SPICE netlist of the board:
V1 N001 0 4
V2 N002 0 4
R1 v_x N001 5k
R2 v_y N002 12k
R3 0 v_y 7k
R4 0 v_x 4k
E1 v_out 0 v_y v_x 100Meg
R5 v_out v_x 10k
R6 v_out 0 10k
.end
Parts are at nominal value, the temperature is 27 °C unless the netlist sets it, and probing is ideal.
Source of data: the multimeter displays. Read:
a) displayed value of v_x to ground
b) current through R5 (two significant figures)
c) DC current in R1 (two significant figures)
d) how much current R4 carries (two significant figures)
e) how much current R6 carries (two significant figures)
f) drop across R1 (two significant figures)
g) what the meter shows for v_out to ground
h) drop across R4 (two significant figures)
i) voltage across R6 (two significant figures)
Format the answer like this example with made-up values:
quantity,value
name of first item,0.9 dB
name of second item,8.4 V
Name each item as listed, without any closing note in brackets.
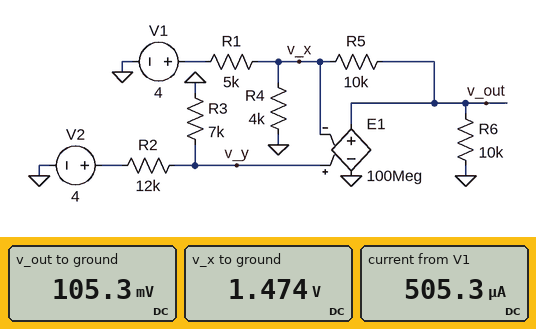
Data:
quantity,value
displayed value of v_x to ground,1.474 V
current through R5,140 µA
DC current in R1,510 µA
how much current R4 carries,370 µA
how much current R6 carries,11 µA
drop across R1,2.5 V
what the meter shows for v_out to ground,105.3 mV
drop across R4,1.5 V
voltage across R6,110 mV
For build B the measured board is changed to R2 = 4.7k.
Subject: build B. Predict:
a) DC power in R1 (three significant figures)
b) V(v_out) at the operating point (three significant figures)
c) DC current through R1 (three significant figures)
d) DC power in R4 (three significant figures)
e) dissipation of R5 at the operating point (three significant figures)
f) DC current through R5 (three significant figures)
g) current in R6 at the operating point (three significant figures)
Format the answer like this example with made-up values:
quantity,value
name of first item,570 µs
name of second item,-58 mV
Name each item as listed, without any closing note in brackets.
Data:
quantity,value
DC power in R1,516 µW
V(v_out) at the operating point,5.16 V
DC current through R1,321 µA
DC power in R4,1.43 mW
dissipation of R5 at the operating point,767 µW
DC current through R5,277 µA
current in R6 at the operating point,516 µA
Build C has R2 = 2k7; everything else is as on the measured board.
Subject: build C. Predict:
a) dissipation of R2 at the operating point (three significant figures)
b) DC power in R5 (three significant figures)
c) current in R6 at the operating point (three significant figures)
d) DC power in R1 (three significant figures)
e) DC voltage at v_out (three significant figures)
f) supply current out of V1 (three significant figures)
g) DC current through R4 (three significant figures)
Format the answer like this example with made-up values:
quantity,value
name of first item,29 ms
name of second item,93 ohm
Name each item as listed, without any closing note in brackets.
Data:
quantity,value
dissipation of R2 at the operating point,459 µW
DC power in R5,2.49 mW
current in R6 at the operating point,788 µA
DC power in R1,248 µW
DC voltage at v_out,7.88 V
supply current out of V1,223 µA
DC current through R4,722 µA
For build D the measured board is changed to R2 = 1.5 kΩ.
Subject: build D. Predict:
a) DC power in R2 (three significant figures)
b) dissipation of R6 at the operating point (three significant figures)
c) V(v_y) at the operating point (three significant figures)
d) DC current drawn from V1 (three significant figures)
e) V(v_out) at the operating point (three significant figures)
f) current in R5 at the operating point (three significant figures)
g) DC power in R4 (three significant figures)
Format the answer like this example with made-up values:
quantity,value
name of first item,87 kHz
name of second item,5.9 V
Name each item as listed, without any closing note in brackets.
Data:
quantity,value
DC power in R2,332 µW
dissipation of R6 at the operating point,10.2 mW
V(v_y) at the operating point,3.29 V
DC current drawn from V1,141 µA
V(v_out) at the operating point,10.1 V
current in R5 at the operating point,682 µA
DC power in R4,2.71 mW
